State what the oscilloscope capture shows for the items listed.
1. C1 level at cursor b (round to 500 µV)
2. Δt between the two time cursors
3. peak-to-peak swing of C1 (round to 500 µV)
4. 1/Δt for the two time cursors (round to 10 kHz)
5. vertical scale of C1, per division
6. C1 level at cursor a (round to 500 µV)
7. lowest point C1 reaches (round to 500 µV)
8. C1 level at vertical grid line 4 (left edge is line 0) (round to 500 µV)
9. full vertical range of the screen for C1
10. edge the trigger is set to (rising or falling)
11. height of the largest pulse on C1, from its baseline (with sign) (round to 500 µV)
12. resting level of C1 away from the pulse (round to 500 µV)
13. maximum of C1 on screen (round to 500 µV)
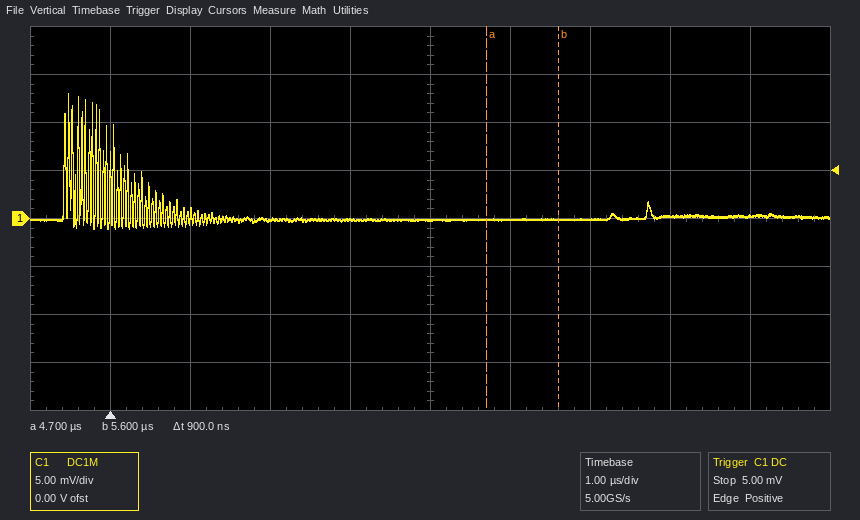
0.0 mV
900 ns
14.0 mV
1.11 MHz
5 mV
0.0 mV
-1.0 mV
0.0 mV
40 mV
rising
+13.0 mV
0.0 mV
13.0 mV
